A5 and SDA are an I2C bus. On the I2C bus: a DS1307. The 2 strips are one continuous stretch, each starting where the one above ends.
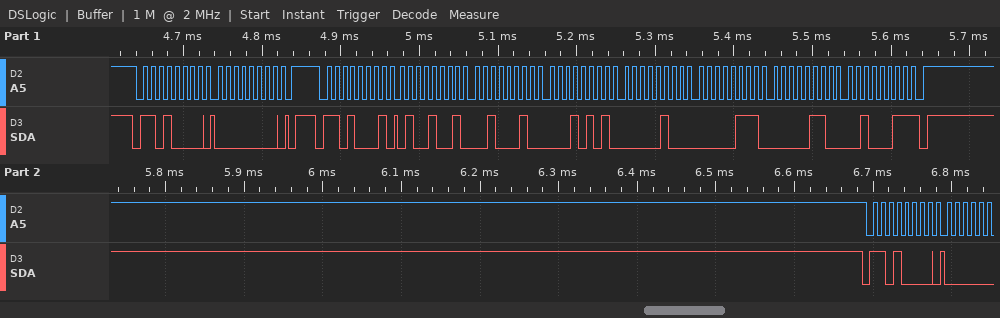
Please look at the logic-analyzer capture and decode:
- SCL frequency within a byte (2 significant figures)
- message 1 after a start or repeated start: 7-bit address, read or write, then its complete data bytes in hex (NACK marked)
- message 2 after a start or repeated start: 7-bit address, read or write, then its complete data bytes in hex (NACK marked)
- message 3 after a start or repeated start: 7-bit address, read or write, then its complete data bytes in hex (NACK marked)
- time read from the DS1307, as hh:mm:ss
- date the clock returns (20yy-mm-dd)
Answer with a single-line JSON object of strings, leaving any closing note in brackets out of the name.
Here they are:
{"SCL frequency within a byte": "100 kHz", "message 1 after a start or repeated start: 7-bit address, read or write, then its complete data bytes in hex": "0x68 write: 00", "message 2 after a start or repeated start: 7-bit address, read or write, then its complete data bytes in hex": "0x68 read: 49 22 15 04 07 06 23 NACK", "message 3 after a start or repeated start: 7-bit address, read or write, then its complete data bytes in hex": "0x68 write", "time read from the DS1307, as hh:mm:ss": "15:22:49", "date the clock returns": "2023-06-07"}
